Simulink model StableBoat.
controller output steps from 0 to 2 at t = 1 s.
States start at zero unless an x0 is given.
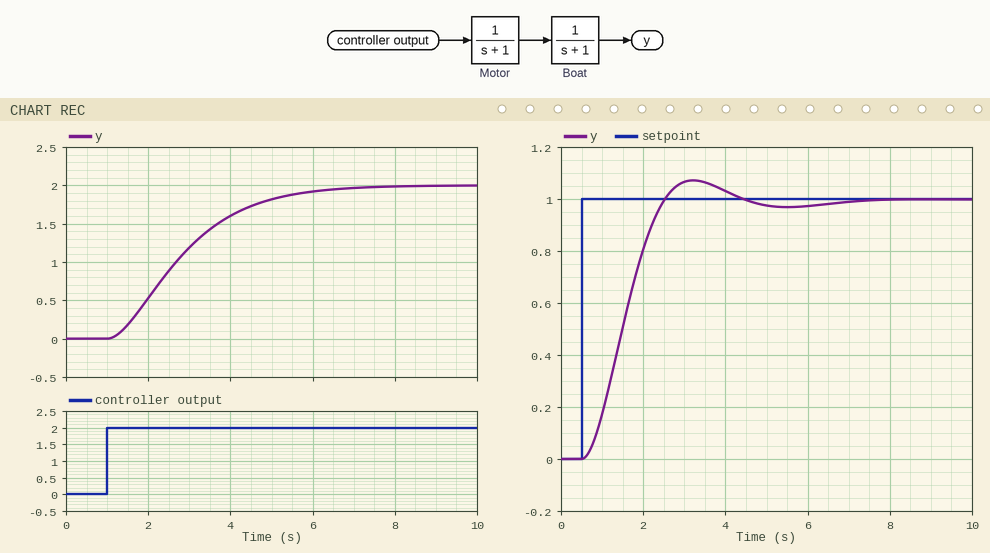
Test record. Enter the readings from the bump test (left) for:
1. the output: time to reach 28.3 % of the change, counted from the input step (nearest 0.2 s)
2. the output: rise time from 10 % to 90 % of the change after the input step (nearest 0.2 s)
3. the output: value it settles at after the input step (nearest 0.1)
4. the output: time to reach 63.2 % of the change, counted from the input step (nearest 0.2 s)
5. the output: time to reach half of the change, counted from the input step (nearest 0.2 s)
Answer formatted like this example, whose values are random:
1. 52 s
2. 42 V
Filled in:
1. 1.0 s
2. 3.4 s
3. 2.0
4. 2.2 s
5. 1.6 s
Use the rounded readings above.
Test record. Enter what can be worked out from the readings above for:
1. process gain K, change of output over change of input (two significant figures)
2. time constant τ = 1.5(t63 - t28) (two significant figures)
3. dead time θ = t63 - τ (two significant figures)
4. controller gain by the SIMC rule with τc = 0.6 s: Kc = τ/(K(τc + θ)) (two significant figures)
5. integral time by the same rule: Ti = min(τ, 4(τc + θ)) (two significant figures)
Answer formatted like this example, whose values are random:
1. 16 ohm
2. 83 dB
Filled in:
1. 1.0
2. 1.8 s
3. 0.40 s
4. 1.8
5. 1.8 s
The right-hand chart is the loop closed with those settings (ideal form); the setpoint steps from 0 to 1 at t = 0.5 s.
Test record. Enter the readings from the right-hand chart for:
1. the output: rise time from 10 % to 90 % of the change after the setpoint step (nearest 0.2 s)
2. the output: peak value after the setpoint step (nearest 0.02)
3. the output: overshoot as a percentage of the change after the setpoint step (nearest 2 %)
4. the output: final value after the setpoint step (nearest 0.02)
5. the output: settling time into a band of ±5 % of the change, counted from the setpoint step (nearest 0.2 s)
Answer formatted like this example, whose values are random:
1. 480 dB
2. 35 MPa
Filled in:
1. 1.4 s
2. 1.08
3. 8 %
4. 1.00
5. 3.2 s
